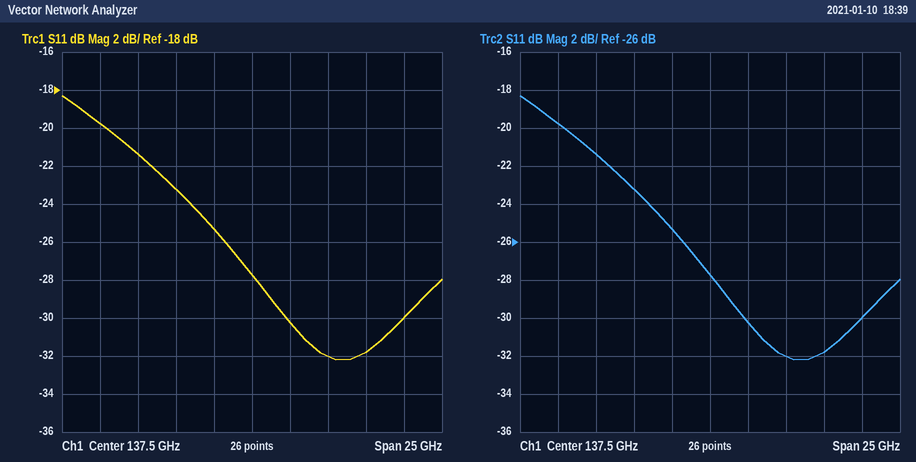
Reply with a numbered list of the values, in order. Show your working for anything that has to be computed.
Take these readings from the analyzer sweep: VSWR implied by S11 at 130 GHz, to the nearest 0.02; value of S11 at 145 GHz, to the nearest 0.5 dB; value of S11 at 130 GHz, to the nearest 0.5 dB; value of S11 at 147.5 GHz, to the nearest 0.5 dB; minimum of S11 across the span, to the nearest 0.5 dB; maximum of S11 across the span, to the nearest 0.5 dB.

1. |Γ| = 10^(-21.5/20) = 0.0841; VSWR = (1 + 0.0841)/(1 − 0.0841) ≈ 1.18
2. -32.0 dB
3. -21.5 dB
4. -30.0 dB
5. -32.0 dB
6. -18.5 dB
